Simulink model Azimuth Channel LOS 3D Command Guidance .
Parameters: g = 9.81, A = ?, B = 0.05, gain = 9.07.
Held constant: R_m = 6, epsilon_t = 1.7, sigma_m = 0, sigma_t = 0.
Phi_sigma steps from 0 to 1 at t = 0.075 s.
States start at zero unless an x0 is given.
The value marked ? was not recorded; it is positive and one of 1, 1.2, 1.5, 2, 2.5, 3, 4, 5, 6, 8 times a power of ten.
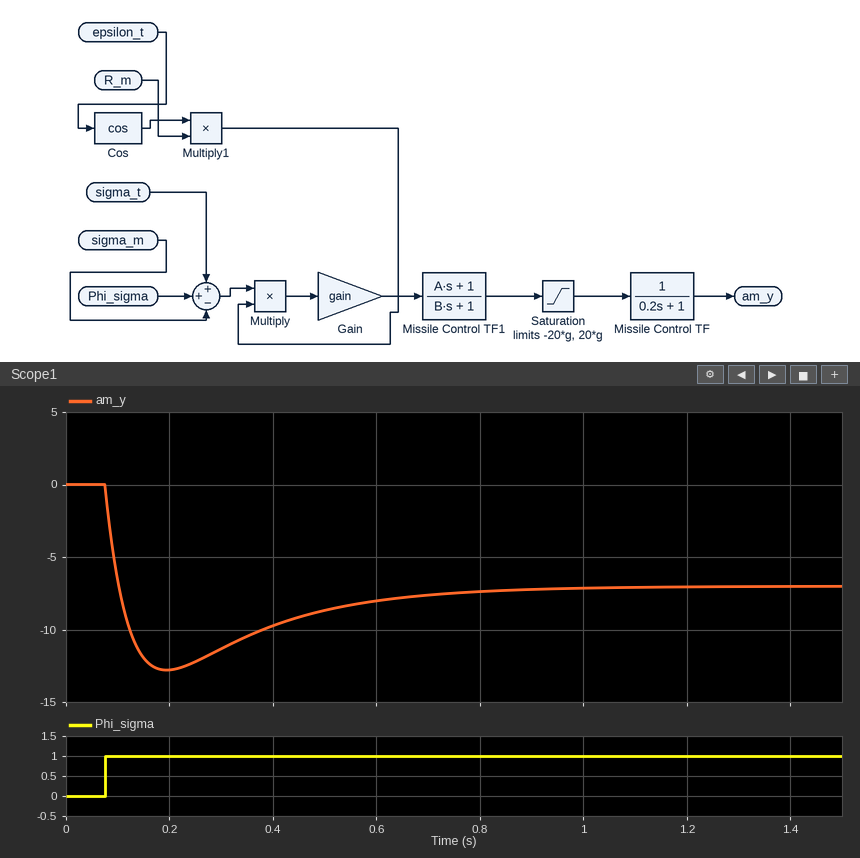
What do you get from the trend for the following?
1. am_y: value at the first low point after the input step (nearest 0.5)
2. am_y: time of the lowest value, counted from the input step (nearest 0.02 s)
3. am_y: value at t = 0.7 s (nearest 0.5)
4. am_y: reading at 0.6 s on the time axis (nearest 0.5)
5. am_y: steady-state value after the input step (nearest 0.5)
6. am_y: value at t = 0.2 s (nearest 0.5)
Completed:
-13.0
0.12 s
-7.5
-8.0
-7.0
-13.0
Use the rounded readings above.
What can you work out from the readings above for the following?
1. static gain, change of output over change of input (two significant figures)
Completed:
-7.0
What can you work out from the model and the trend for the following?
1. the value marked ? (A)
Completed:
0.5
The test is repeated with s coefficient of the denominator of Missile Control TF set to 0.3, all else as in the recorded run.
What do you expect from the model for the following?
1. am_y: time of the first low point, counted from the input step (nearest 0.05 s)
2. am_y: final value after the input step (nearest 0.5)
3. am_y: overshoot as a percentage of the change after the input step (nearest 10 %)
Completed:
0.15 s
-7.0
40 %
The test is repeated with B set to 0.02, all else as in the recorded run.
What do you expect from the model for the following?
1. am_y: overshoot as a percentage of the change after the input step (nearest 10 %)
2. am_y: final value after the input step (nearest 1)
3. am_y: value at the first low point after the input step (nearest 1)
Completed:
110 %
-7
-15
